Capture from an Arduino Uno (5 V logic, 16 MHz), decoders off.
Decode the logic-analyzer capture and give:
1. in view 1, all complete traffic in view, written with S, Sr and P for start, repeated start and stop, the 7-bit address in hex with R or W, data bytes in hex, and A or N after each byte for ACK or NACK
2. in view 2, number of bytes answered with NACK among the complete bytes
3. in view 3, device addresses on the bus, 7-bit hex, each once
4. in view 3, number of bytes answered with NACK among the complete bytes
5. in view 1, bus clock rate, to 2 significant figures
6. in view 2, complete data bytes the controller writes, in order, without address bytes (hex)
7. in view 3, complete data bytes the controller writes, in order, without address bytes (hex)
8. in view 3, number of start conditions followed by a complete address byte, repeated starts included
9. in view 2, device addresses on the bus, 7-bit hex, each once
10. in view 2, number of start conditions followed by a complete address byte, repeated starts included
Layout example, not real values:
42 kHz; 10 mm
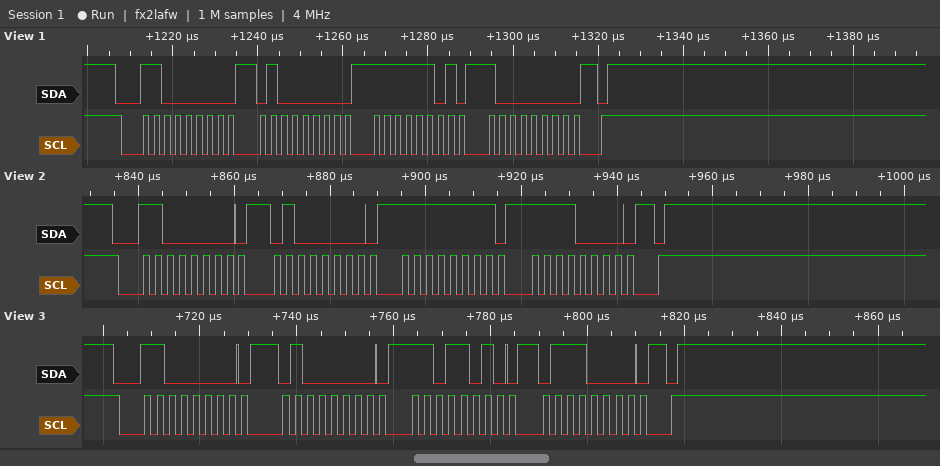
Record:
S 60W A 40 A FD A 80 A P; 0; 0x60; 0; 400 kHz; 40 FF F0; 40 DA 70; 1; 0x60; 1
